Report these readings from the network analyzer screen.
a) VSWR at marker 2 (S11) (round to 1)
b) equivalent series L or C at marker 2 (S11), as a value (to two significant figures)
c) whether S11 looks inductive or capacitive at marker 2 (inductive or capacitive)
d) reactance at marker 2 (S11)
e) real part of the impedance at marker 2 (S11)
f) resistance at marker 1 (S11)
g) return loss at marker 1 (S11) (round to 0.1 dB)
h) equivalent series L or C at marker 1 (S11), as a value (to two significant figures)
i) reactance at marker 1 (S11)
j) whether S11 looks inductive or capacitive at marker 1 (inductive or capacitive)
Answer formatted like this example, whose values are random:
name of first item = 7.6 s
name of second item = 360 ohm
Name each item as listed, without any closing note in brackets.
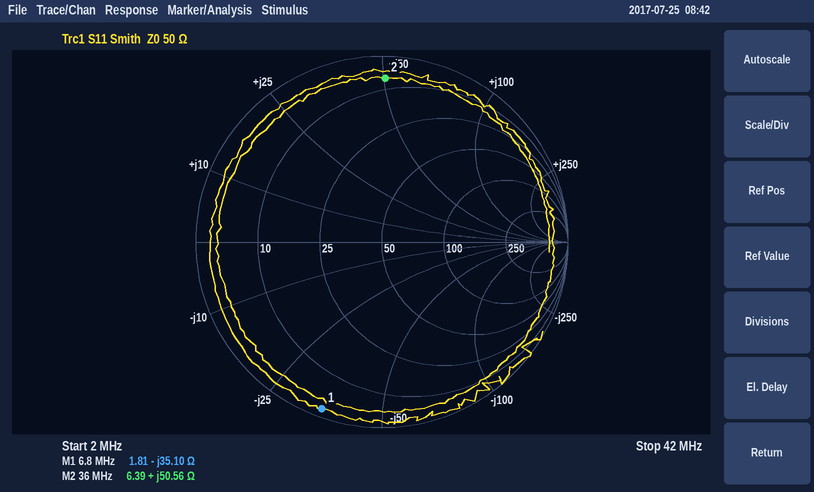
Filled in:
VSWR at marker 2 (S11) = 16
equivalent series L or C at marker 2 (S11), as a value = 220 nH
whether S11 looks inductive or capacitive at marker 2 = inductive
reactance at marker 2 = +50.56 Ω
real part of the impedance at marker 2 = 6.39 Ω
resistance at marker 1 = 1.81 Ω
return loss at marker 1 (S11) = 0.4 dB
equivalent series L or C at marker 1 (S11), as a value = 670 pF
reactance at marker 1 = -35.10 Ω
whether S11 looks inductive or capacitive at marker 1 = capacitive
